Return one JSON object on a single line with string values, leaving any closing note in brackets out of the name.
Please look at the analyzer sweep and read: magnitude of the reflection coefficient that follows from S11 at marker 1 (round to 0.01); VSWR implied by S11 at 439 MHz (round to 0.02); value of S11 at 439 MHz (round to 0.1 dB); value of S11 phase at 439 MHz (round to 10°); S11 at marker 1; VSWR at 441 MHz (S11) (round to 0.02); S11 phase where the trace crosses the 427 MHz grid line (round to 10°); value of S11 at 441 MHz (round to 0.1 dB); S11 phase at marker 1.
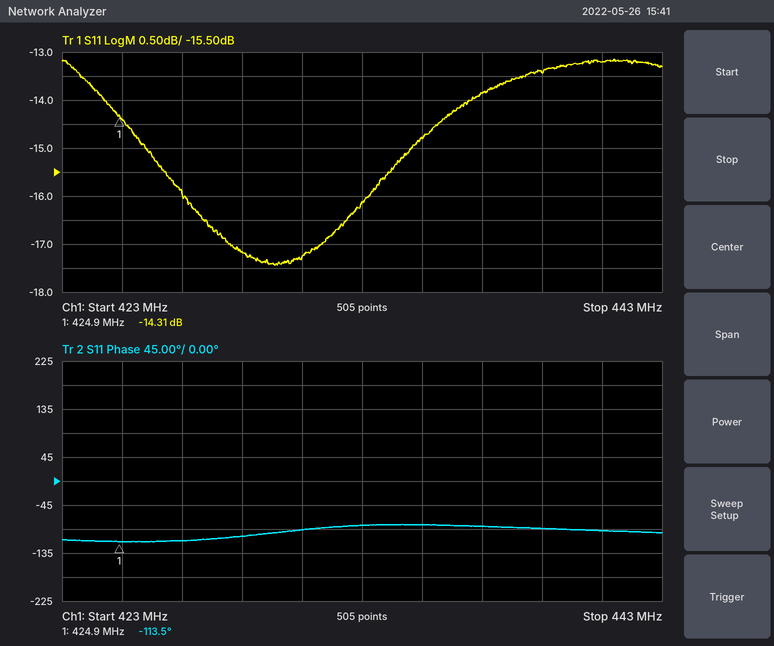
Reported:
{"magnitude of the reflection coefficient that follows from S11 at marker 1": "0.19", "VSWR implied by S11 at 439 MHz": "1.54", "value of S11 at 439 MHz": "-13.4 dB", "value of S11 phase at 439 MHz": "-90°", "S11 at marker 1": "-14.31 dB", "VSWR at 441 MHz (S11)": "1.56", "S11 phase where the trace crosses the 427 MHz grid line": "-110°", "value of S11 at 441 MHz": "-13.2 dB", "S11 phase at marker 1": "-113.5°"}
